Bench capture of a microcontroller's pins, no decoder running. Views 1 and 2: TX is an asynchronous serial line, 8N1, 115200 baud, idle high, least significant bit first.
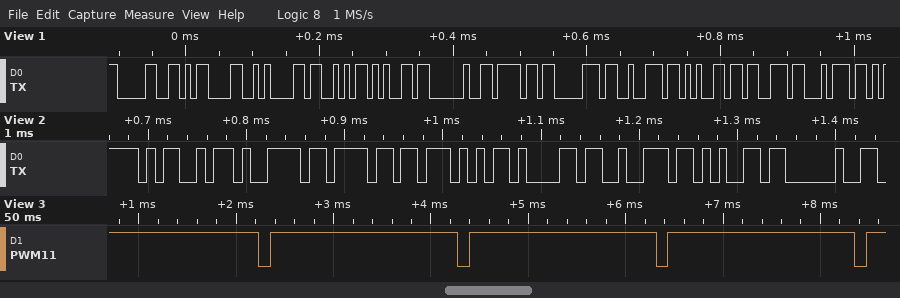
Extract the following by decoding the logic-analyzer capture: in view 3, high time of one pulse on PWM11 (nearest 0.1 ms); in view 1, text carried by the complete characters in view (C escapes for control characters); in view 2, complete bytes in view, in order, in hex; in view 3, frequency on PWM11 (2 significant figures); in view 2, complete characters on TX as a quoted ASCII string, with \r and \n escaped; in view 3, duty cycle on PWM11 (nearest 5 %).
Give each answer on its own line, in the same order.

1.9 ms
"0\r\nSe oprest"
4D 79 6F 57 61 72 65 20
490 Hz
"MyoWare "
95 %
